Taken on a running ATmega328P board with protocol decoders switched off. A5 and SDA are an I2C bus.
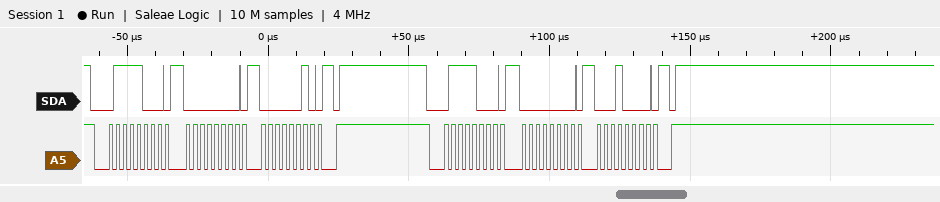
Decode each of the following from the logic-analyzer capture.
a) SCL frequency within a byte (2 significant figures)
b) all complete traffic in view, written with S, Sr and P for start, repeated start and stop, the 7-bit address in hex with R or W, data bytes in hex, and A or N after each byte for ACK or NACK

400 kHz
S 3CW A 00 A 02 A P S 3CW A 00 A 10 A P
